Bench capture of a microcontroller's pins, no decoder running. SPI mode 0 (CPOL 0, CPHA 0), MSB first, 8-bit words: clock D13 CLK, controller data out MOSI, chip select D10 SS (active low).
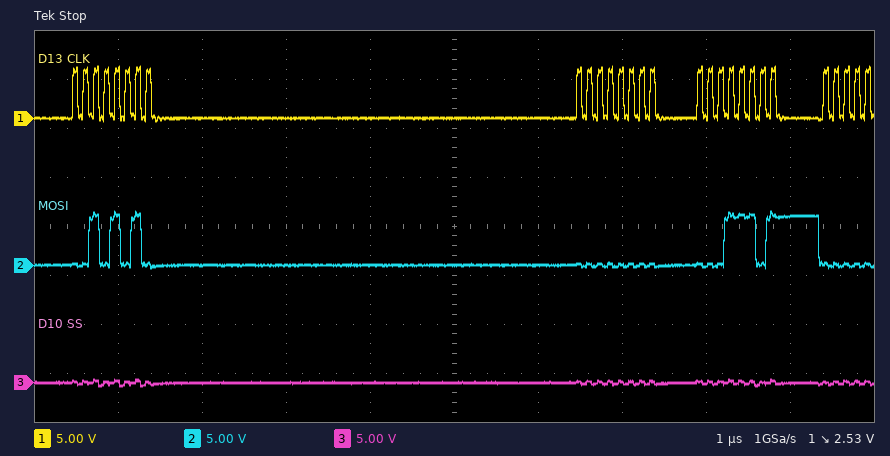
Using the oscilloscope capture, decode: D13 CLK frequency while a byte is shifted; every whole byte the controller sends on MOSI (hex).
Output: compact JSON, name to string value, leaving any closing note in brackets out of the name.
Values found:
{"D13 CLK frequency while a byte is shifted": "8 MHz", "every whole byte the controller sends on MOSI": "2A 00 1D"}
